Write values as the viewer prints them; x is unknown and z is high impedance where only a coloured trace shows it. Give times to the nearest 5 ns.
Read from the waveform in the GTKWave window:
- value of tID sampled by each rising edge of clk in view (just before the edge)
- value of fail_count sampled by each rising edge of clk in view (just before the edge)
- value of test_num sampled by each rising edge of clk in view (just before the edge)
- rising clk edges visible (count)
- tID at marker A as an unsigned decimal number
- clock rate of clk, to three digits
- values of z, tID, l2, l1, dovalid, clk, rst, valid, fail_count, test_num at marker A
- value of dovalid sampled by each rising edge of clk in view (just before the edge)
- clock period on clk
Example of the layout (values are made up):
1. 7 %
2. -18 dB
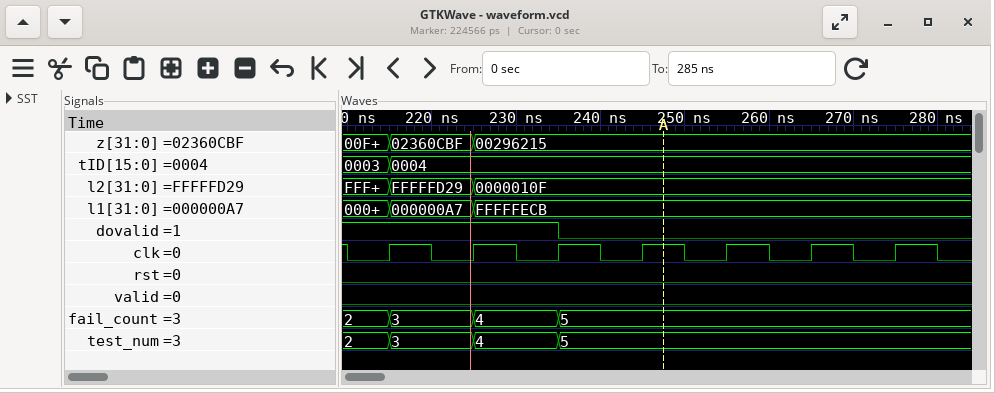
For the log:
1. 0003, 0004, 0004, 0004, 0004, 0004, 0004
2. 2, 3, 4, 5, 5, 5, 5
3. 2, 3, 4, 5, 5, 5, 5
4. 7
5. 4
6. 100 MHz
7. z=00296215, tID=0004, l2=0000010F, l1=FFFFFECB, dovalid=0, clk=1, rst=0, valid=0, fail_count=5, test_num=5
8. 1 1 1 0 0 0 0
9. 10 ns
